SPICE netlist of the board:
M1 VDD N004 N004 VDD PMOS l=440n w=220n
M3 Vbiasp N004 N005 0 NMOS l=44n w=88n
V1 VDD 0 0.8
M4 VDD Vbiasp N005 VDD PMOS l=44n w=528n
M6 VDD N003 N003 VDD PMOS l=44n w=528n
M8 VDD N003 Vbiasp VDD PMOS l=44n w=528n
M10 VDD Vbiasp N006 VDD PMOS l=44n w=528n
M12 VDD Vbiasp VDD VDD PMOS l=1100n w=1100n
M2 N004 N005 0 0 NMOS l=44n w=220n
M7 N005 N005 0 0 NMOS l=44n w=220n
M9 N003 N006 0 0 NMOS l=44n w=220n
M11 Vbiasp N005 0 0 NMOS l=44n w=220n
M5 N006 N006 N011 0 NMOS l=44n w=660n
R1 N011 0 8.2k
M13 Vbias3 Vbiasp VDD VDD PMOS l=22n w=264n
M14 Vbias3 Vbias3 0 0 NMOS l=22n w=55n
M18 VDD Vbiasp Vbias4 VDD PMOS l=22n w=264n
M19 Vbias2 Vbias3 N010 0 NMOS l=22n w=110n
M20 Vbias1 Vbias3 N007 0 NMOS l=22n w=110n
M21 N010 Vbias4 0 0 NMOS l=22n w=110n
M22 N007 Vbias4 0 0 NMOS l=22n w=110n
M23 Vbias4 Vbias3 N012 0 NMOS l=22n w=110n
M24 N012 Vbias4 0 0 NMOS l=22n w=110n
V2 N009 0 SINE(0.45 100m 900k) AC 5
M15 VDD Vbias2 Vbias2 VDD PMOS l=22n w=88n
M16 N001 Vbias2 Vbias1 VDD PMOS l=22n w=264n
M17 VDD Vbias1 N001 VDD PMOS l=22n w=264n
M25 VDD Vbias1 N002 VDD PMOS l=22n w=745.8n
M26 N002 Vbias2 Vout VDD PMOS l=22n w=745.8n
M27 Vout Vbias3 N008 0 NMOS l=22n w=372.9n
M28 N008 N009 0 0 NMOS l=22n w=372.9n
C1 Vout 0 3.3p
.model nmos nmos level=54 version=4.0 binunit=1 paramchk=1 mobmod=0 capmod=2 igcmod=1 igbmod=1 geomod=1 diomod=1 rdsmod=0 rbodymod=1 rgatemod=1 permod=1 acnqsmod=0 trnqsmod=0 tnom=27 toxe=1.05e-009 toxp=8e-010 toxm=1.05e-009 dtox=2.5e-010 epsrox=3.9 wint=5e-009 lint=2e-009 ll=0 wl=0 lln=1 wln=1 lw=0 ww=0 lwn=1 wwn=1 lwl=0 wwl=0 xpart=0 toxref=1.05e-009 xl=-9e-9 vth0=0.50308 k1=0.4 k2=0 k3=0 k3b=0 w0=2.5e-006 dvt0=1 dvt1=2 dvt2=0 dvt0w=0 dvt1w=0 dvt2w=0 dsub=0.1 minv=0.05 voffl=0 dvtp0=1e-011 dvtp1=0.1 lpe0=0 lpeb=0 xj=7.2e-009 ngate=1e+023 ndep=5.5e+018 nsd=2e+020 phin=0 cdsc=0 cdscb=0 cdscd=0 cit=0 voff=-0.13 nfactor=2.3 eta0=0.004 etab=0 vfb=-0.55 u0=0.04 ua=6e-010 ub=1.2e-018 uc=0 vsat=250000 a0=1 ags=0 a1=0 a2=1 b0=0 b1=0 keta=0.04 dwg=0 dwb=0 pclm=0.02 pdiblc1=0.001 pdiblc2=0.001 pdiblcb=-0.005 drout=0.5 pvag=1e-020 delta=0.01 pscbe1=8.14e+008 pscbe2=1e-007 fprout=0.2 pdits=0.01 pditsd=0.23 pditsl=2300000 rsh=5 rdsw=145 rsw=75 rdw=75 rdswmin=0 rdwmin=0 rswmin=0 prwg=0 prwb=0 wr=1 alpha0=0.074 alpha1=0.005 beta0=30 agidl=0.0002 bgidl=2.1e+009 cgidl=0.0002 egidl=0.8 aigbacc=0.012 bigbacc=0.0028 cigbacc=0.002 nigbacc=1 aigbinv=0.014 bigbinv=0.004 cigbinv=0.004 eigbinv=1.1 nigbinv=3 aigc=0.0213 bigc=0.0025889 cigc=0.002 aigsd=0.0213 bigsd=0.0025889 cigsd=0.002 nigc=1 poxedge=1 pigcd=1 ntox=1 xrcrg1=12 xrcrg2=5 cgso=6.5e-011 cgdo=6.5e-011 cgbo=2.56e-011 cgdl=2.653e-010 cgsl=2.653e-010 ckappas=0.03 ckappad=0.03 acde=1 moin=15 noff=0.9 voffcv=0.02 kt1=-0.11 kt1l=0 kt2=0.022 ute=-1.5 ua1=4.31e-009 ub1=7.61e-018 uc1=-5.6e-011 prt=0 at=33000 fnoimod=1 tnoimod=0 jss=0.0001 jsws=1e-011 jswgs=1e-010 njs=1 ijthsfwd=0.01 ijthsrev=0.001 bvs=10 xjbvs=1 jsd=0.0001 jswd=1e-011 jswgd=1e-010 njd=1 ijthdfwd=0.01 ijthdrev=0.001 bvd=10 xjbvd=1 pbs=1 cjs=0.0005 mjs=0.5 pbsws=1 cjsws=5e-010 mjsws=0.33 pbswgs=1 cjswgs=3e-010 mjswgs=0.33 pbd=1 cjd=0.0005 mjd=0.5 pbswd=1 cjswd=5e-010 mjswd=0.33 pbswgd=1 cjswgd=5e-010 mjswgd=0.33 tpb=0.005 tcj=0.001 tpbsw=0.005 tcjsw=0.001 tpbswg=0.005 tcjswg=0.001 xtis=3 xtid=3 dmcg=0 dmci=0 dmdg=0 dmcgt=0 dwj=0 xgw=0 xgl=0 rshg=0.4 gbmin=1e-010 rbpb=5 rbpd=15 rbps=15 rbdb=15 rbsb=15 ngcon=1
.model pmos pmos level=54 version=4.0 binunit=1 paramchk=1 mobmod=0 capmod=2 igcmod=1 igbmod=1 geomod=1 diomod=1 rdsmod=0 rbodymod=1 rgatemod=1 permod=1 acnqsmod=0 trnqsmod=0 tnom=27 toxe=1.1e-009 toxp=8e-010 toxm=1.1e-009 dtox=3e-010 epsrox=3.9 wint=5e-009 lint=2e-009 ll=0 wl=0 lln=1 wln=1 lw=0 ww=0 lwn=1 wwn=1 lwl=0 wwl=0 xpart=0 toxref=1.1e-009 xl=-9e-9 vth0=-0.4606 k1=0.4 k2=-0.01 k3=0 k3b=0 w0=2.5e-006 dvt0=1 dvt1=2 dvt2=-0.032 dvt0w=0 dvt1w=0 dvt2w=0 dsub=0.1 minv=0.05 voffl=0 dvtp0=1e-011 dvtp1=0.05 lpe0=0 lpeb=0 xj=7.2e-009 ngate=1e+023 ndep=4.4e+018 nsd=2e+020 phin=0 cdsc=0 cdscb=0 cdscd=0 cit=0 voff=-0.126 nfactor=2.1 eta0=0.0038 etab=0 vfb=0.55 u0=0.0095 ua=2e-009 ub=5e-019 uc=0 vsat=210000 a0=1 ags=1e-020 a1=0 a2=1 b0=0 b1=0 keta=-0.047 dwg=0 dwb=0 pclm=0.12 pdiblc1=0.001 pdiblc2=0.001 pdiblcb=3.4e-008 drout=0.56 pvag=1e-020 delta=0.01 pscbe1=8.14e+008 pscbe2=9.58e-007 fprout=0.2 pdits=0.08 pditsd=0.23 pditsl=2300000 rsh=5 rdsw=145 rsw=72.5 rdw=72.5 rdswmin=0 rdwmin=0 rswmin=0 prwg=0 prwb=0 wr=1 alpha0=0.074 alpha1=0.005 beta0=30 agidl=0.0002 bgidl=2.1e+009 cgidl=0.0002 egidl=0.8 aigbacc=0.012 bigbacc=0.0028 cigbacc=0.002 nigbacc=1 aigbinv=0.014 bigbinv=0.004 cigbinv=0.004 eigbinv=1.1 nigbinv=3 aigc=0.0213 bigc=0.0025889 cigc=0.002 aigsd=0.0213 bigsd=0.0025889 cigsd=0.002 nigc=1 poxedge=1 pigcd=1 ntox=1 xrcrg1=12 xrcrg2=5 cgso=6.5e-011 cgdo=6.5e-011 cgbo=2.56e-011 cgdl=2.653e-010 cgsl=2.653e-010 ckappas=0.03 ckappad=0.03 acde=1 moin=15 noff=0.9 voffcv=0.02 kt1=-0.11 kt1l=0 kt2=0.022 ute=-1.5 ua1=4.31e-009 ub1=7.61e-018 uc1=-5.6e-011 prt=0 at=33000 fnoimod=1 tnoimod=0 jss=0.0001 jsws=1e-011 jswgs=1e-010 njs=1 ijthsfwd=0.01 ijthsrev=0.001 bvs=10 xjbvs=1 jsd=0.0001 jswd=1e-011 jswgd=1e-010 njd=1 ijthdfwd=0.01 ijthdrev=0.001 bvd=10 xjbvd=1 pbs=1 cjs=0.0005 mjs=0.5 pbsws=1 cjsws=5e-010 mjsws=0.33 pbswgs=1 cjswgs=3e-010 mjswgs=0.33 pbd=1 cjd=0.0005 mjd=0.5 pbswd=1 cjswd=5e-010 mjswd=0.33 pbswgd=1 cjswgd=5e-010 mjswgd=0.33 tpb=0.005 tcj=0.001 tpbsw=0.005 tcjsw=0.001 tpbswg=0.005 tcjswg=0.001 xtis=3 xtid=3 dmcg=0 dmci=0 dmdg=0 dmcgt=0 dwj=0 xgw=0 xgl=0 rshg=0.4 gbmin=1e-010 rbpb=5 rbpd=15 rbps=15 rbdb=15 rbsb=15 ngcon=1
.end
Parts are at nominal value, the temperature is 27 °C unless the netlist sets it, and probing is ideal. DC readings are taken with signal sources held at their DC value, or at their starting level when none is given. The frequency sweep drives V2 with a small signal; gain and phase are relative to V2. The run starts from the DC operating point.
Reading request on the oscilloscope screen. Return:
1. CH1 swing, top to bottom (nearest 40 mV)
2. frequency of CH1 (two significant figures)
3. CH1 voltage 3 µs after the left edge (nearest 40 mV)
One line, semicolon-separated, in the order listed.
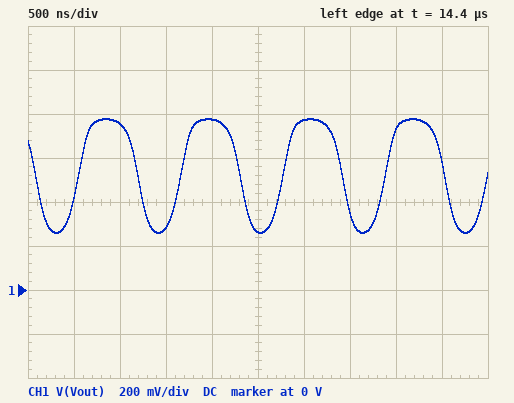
520 mV; 900 kHz; 760 mV
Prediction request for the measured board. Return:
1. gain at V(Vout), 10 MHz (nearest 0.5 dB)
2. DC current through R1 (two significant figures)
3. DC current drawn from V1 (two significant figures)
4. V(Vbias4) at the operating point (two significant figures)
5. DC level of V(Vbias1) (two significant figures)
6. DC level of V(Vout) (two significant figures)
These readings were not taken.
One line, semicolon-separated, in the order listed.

3.0 dB; 5.9 µA; 130 µA; 610 mV; 260 mV; 630 mV
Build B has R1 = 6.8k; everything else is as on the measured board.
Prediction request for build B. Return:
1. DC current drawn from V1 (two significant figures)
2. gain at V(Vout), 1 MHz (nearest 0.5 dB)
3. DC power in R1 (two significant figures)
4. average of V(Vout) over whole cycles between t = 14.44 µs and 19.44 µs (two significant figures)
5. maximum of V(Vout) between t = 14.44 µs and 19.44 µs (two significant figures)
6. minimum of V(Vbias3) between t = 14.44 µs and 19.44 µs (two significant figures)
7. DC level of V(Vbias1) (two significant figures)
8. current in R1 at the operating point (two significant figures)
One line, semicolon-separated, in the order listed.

150 µA; 10.5 dB; 370 nW; 570 mV; 780 mV; 590 mV; 250 mV; 7.4 µA
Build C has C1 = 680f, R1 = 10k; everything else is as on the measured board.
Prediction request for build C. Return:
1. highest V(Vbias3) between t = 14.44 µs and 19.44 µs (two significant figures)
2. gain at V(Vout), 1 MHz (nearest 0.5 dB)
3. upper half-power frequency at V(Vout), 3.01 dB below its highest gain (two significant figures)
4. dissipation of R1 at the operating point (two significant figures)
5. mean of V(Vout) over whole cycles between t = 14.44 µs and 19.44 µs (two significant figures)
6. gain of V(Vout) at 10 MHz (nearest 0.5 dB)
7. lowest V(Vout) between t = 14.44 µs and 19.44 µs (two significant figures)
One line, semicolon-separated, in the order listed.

560 mV; 12.0 dB; 17 MHz; 220 nW; 550 mV; 11.0 dB; 250 mV
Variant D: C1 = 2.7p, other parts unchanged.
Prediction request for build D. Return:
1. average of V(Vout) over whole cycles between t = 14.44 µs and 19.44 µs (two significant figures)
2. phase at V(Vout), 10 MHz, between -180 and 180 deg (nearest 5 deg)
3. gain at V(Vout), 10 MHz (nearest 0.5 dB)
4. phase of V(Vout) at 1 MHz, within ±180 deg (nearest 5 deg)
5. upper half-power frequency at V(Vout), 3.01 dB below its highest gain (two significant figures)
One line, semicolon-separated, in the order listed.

560 mV; 115 deg; 4.5 dB; 170 deg; 4.8 MHz
